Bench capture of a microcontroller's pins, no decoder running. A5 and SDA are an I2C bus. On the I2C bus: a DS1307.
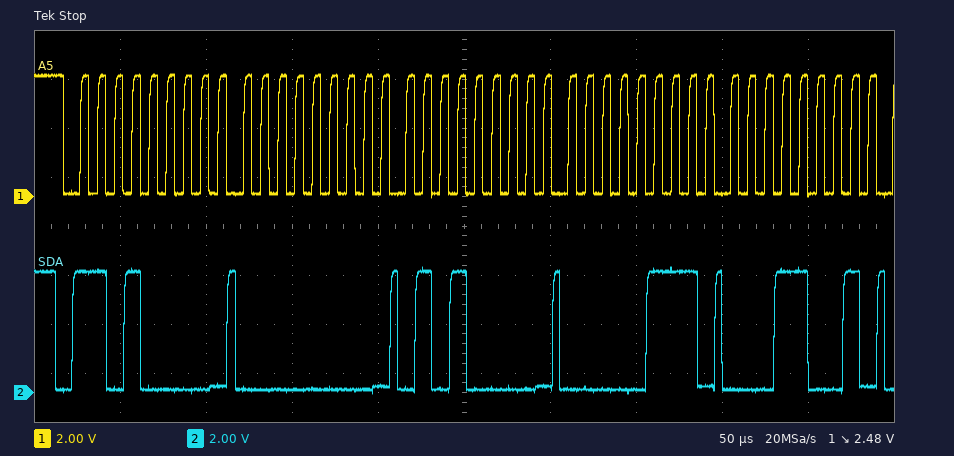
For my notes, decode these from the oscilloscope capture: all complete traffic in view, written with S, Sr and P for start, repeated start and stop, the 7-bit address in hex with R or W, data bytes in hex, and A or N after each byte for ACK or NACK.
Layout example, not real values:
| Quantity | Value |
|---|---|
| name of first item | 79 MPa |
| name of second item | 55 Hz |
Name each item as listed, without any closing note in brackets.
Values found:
| Quantity | Value |
|---|---|
| all complete traffic in view, written with S, Sr and P for start, repeated start and stop, the 7-bit address in hex with R or W, data bytes in hex, and A or N after each byte for ACK or NACK | S 68W A 00 A 50 A 07 A 19 A |
